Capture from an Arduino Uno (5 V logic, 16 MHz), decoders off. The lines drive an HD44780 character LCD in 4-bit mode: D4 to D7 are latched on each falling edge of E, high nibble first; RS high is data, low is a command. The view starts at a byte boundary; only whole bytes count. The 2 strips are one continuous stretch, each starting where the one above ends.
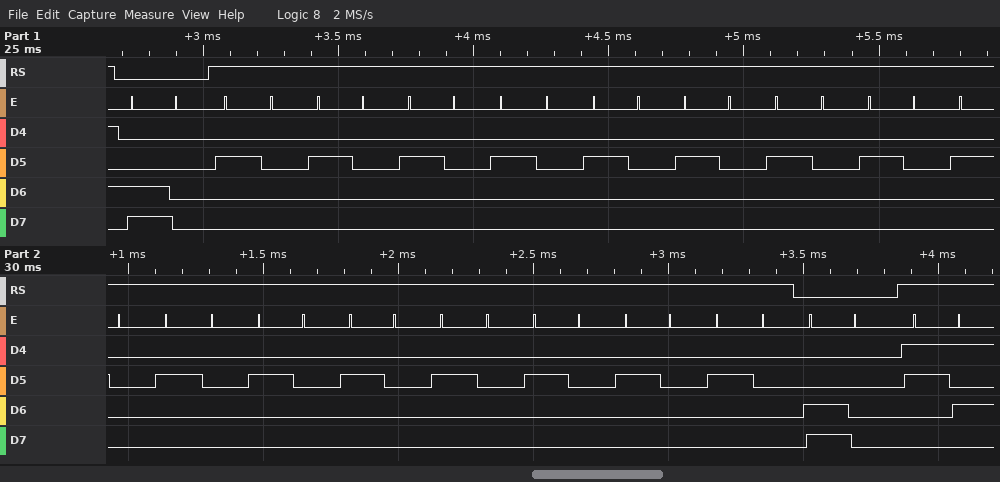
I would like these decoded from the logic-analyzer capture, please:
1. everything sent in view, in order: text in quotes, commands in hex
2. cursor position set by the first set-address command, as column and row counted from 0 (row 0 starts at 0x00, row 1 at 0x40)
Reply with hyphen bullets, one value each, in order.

- 0xC0 "                " 0xC0 "5"
- column 0, row 1
